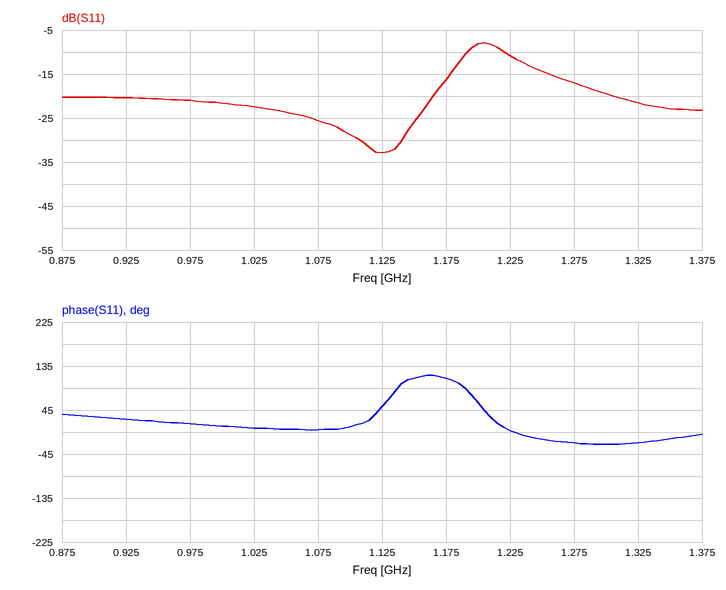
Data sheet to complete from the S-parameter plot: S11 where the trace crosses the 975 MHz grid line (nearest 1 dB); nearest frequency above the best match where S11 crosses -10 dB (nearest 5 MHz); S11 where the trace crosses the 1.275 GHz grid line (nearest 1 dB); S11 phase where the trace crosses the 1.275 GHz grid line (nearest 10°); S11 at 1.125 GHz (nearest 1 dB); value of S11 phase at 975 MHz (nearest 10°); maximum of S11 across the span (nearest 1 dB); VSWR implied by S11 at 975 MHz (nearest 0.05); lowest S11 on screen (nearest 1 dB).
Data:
-21 dB
1.190 GHz
-17 dB
-20°
-33 dB
20°
-8 dB
1.20
-33 dB
